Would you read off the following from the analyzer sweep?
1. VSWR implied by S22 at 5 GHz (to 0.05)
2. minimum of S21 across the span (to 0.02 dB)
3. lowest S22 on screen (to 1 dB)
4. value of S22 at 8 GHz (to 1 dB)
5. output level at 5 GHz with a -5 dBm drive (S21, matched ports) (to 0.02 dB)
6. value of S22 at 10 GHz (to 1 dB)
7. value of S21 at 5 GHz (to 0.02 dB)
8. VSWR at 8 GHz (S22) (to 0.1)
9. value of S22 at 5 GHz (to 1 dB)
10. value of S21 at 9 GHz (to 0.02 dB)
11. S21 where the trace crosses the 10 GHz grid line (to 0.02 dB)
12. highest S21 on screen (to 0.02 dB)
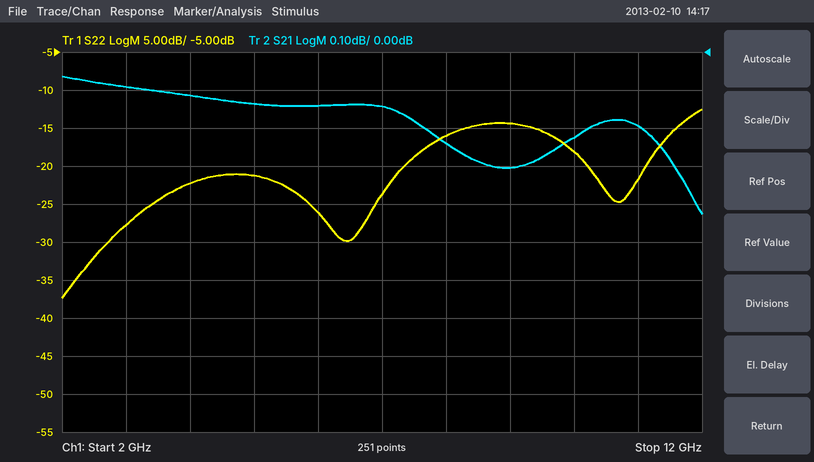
1.20
-0.42 dB
-37 dB
-16 dB
-5.14 dBm
-18 dB
-0.14 dB
1.4
-21 dB
-0.30 dB
-0.22 dB
-0.06 dB
